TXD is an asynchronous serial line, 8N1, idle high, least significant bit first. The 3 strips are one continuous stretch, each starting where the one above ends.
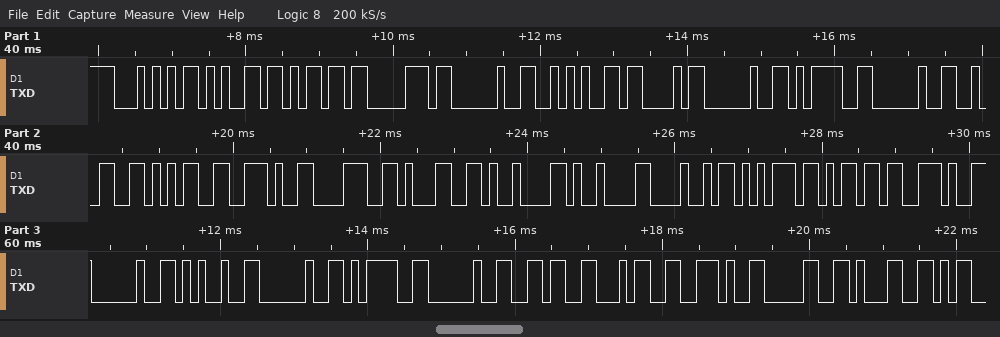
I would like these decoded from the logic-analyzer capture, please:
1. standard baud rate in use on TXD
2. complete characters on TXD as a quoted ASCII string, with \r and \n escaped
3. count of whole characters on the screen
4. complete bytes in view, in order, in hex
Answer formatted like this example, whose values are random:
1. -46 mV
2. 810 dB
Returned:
1. 9600 baud
2. "Temp *C = 25.81\t\tHum. % = 64.01"
3. 31
4. 54 65 6D 70 20 2A 43 20 3D 20 32 35 2E 38 31 09 09 48 75 6D 2E 20 25 20 3D 20 36 34 2E 30 31
